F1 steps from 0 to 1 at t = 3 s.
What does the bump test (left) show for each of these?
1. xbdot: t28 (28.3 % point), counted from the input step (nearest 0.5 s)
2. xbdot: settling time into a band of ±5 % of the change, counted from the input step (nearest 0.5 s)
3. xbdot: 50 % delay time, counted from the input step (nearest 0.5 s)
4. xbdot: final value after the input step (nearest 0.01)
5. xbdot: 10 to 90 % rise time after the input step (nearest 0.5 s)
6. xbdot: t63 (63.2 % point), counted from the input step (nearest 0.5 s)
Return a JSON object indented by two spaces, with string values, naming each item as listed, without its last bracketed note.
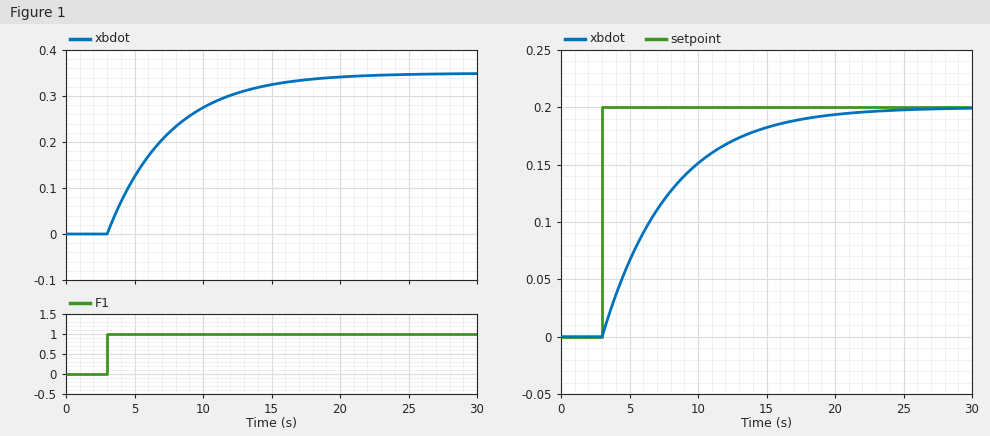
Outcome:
{
  "xbdot: t28 (28.3 % point), counted from the input step": "1.5 s",
  "xbdot: settling time into a band of ±5 % of the change, counted from the input step": "13.5 s",
  "xbdot: 50 % delay time, counted from the input step": "3.0 s",
  "xbdot: final value after the input step": "0.35",
  "xbdot: 10 to 90 % rise time after the input step": "10.0 s",
  "xbdot: t63 (63.2 % point), counted from the input step": "4.5 s"
}
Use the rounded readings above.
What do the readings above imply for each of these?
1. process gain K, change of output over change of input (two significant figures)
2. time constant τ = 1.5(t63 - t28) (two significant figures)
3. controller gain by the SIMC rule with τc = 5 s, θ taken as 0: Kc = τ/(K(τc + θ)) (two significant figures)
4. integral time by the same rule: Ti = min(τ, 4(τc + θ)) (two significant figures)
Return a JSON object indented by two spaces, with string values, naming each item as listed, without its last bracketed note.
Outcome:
{
  "process gain K, change of output over change of input": "0.35",
  "time constant τ = 1.5(t63 - t28)": "4.5 s",
  "controller gain by the SIMC rule with τc = 5 s, θ taken as 0: Kc = τ/(K(τc + θ))": "2.6",
  "integral time by the same rule: Ti = min(τ, 4(τc + θ))": "4.5 s"
}
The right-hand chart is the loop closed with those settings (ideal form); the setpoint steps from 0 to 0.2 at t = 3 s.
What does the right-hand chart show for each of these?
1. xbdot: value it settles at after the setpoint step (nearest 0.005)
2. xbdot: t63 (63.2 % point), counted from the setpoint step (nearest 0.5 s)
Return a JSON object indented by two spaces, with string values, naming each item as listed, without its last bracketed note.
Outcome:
{
  "xbdot: value it settles at after the setpoint step": "0.200",
  "xbdot: t63 (63.2 % point), counted from the setpoint step": "5.0 s"
}
